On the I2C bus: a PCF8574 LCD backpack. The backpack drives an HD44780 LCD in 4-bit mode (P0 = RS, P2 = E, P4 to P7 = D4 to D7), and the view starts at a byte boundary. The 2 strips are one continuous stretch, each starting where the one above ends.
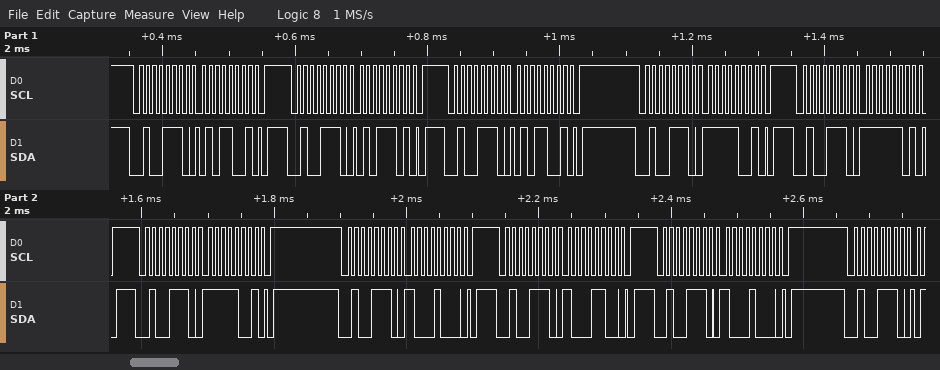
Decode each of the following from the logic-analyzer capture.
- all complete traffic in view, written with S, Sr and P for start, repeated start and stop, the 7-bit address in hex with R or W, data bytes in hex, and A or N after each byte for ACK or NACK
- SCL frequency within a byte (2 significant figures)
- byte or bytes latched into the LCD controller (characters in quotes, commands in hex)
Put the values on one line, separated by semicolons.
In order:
S 27W A 59 A P S 27W A 5D A P S 27W A 59 A P S 27W A F9 A P S 27W A FD A P S 27W A F9 A P S 27W A 88 A P S 27W A 8C A P S 27W A 88 A P S 27W A; 100 kHz; '_'
